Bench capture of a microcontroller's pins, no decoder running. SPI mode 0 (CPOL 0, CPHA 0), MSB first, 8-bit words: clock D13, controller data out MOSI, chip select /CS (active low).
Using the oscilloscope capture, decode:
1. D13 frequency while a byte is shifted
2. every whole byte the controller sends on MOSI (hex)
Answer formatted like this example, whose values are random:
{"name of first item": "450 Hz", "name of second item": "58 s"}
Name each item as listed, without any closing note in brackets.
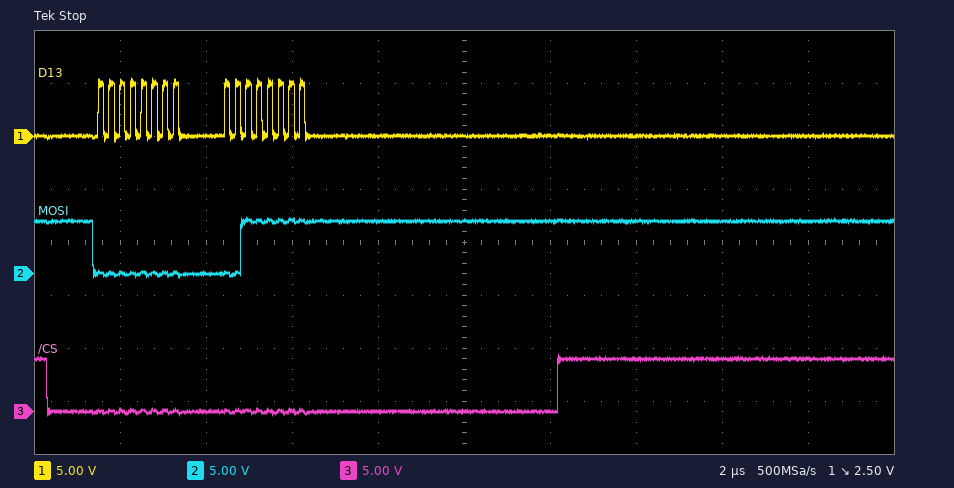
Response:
{"D13 frequency while a byte is shifted": "4 MHz", "every whole byte the controller sends on MOSI": "00 3F"}
